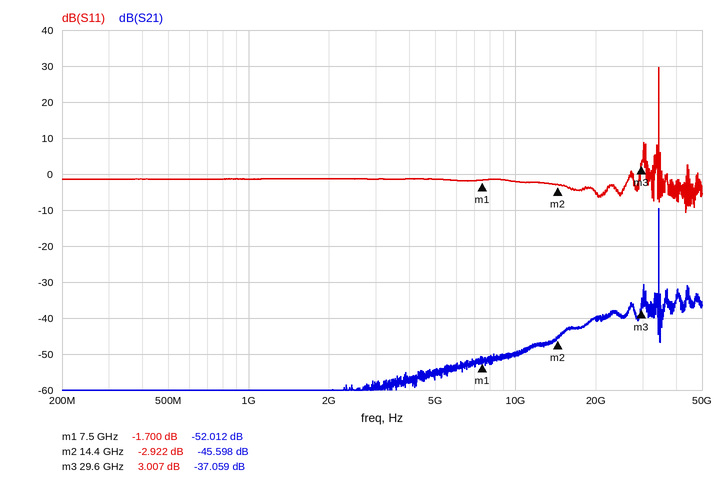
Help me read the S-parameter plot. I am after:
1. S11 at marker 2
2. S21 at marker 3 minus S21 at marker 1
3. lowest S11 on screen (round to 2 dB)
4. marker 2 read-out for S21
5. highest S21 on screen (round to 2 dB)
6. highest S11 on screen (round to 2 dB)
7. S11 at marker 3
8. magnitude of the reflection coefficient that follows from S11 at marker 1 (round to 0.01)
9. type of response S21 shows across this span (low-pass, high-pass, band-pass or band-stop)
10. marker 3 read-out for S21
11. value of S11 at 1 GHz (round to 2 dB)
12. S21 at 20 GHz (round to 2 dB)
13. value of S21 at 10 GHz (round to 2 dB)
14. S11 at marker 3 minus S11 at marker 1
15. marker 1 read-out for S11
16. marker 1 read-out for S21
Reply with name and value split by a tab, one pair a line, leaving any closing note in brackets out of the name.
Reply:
S11 at marker 2	-2.922 dB
S21 at marker 3 minus S21 at marker 1	14.953 dB
lowest S11 on screen	-10 dB
marker 2 read-out for S21	-45.598 dB
highest S21 on screen	-10 dB
highest S11 on screen	30 dB
S11 at marker 3	3.007 dB
magnitude of the reflection coefficient that follows from S11 at marker 1	0.82
type of response S21 shows across this span	band-pass
marker 3 read-out for S21	-37.059 dB
value of S11 at 1 GHz	-2 dB
S21 at 20 GHz	-40 dB
value of S21 at 10 GHz	-50 dB
S11 at marker 3 minus S11 at marker 1	4.707 dB
marker 1 read-out for S11	-1.700 dB
marker 1 read-out for S21	-52.012 dB
